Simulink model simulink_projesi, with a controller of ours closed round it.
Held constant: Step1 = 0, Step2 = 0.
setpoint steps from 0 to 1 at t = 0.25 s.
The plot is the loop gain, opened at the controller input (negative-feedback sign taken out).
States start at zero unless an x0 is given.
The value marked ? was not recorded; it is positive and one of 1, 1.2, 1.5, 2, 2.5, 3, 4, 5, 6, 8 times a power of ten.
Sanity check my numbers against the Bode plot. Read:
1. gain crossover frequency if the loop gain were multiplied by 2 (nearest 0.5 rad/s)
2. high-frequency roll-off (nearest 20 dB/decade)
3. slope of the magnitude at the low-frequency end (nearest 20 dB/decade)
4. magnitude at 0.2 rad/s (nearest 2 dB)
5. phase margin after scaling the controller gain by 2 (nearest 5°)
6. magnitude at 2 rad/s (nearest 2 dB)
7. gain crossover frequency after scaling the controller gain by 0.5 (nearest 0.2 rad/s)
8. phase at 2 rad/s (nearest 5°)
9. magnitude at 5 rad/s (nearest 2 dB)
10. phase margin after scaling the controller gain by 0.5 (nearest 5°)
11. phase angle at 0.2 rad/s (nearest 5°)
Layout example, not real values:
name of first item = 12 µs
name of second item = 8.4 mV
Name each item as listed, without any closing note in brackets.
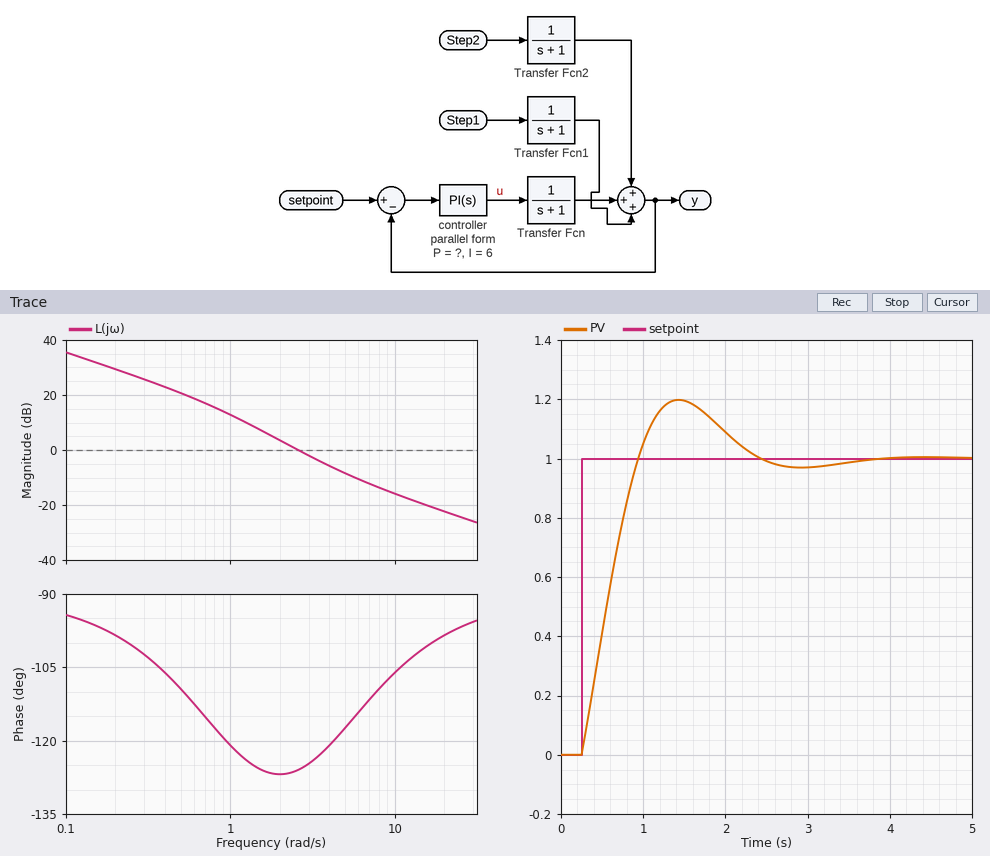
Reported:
gain crossover frequency if the loop gain were multiplied by 2 = 4.0 rad/s
high-frequency roll-off = -20 dB/decade
slope of the magnitude at the low-frequency end = -20 dB/decade
magnitude at 0.2 rad/s = 30 dB
phase margin after scaling the controller gain by 2 = 60°
magnitude at 2 rad/s = 4 dB
gain crossover frequency after scaling the controller gain by 0.5 = 1.6 rad/s
phase at 2 rad/s = -125°
magnitude at 5 rad/s = -8 dB
phase margin after scaling the controller gain by 0.5 = 55°
phase angle at 0.2 rad/s = -100°
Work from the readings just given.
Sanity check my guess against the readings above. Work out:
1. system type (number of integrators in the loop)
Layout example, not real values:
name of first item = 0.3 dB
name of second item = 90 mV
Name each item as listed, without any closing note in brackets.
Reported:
system type = 1
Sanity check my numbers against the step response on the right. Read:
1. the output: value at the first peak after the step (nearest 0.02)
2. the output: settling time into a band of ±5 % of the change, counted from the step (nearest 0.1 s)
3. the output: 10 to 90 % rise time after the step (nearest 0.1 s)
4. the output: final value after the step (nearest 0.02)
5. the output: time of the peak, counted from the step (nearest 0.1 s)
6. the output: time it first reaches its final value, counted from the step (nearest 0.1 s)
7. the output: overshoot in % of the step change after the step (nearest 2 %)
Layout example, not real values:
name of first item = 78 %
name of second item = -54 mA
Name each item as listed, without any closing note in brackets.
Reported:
the output: value at the first peak after the step = 1.20
the output: settling time into a band of ±5 % of the change, counted from the step = 1.9 s
the output: 10 to 90 % rise time after the step = 0.5 s
the output: final value after the step = 1.00
the output: time of the peak, counted from the step = 1.2 s
the output: time it first reaches its final value, counted from the step = 0.7 s
the output: overshoot in % of the step change after the step = 20 %
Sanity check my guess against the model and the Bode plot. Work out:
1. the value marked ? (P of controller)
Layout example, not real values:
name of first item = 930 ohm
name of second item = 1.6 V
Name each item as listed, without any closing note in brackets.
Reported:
the value marked ? = 1.5
